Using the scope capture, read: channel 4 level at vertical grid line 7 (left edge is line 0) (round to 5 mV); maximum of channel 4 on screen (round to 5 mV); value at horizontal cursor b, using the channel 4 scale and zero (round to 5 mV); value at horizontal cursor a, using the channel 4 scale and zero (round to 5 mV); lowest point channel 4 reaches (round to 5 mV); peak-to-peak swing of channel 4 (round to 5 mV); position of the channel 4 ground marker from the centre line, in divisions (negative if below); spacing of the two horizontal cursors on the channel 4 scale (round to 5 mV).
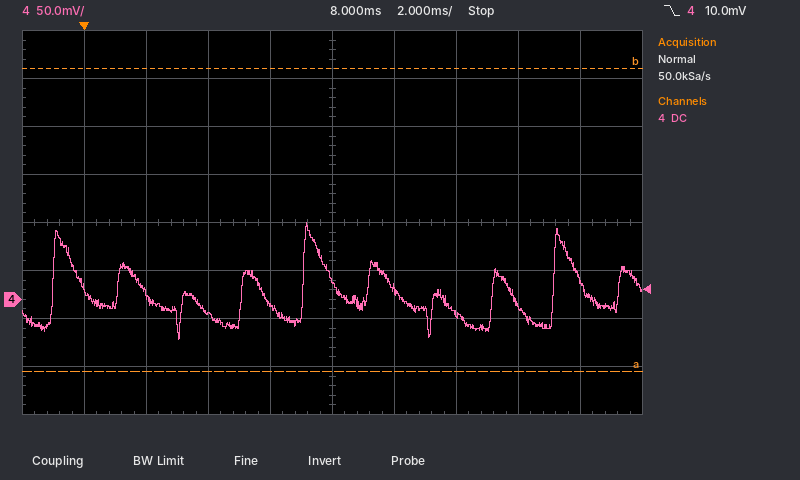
-15 mV
80 mV
240 mV
-75 mV
-40 mV
120 mV
-1.6 div
315 mV
